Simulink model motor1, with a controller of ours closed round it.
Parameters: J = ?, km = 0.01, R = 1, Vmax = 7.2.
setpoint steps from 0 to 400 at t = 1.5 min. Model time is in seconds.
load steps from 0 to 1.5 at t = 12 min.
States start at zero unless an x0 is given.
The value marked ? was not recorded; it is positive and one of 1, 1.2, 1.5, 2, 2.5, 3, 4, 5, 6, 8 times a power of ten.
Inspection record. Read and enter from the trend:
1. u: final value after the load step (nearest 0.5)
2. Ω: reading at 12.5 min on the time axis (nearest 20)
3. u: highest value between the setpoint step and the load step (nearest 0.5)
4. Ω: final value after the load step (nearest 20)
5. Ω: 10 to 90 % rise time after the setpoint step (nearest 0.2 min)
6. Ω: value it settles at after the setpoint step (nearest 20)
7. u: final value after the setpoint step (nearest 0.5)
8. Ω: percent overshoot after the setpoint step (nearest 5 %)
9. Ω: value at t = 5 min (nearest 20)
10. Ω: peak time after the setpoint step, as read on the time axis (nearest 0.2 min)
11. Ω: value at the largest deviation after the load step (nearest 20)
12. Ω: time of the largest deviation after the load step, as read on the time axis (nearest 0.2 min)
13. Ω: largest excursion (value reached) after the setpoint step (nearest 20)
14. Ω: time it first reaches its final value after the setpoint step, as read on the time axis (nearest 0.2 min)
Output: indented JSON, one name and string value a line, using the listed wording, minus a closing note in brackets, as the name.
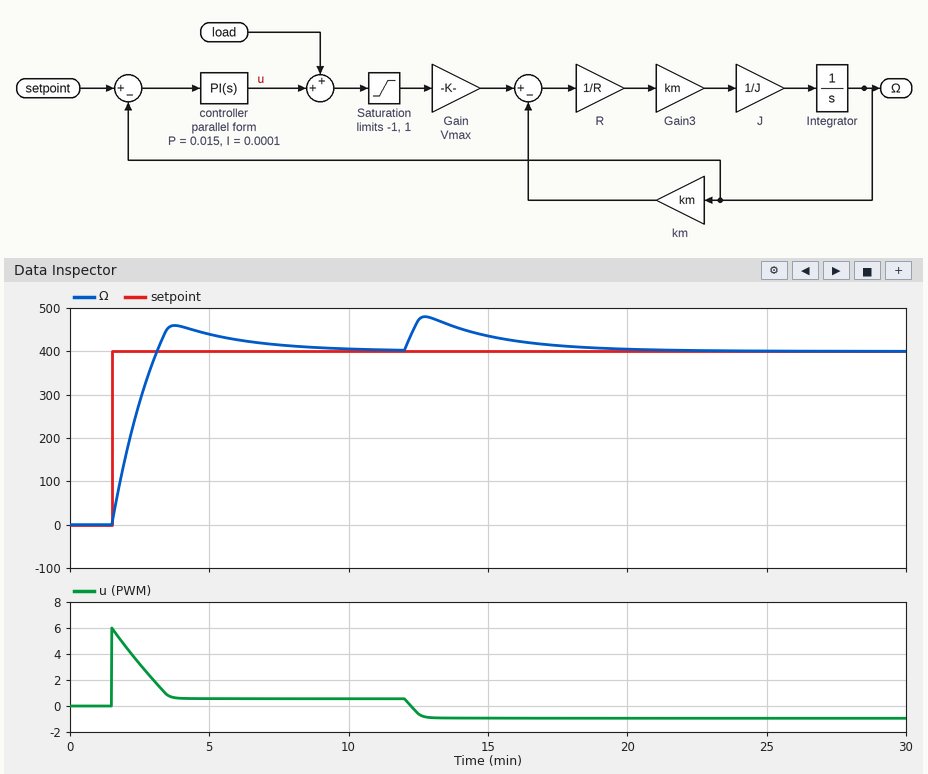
{
  "u: final value after the load step": "-1.0",
  "Ω: reading at 12.5 min on the time axis": "480",
  "u: highest value between the setpoint step and the load step": "6.0",
  "Ω: final value after the load step": "400",
  "Ω: 10 to 90 % rise time after the setpoint step": "1.2 min",
  "Ω: value it settles at after the setpoint step": "400",
  "u: final value after the setpoint step": "0.5",
  "Ω: percent overshoot after the setpoint step": "15 %",
  "Ω: value at t = 5 min": "440",
  "Ω: peak time after the setpoint step, as read on the time axis": "3.8 min",
  "Ω: value at the largest deviation after the load step": "480",
  "Ω: time of the largest deviation after the load step, as read on the time axis": "12.8 min",
  "Ω: largest excursion (value reached) after the setpoint step": "460",
  "Ω: time it first reaches its final value after the setpoint step, as read on the time axis": "3.2 min"
}
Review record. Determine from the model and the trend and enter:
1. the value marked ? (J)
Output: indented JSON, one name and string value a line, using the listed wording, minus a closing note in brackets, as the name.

{
  "the value marked ?": "0.012"
}
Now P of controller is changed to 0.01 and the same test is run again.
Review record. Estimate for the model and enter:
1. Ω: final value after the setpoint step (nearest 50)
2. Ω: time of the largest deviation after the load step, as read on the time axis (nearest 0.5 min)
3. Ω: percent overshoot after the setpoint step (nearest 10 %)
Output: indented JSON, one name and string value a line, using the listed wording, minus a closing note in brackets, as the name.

{
  "Ω: final value after the setpoint step": "400",
  "Ω: time of the largest deviation after the load step, as read on the time axis": "13.0 min",
  "Ω: percent overshoot after the setpoint step": "20 %"
}
